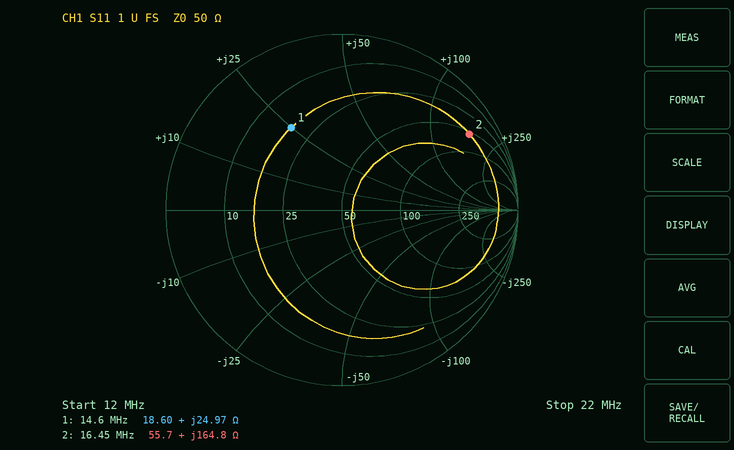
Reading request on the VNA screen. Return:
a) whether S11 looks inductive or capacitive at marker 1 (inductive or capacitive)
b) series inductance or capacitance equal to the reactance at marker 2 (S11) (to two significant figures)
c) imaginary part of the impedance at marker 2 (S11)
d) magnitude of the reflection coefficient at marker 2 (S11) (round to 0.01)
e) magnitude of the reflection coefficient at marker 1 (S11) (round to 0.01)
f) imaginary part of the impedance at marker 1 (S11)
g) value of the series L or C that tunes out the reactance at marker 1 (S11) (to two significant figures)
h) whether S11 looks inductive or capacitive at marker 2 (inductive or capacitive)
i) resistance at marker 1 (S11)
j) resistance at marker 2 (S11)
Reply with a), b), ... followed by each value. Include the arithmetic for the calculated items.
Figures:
a) inductive
b) L = 164.8 Ω/(2π × 16.45 MHz) ≈ 1.6 µH
c) +164.8 Ω
d) 0.84
e) 0.55
f) +24.97 Ω
g) C = 1/(2π × 14.6 MHz × 24.97 Ω) ≈ 437 pF, so 440 pF to two significant figures
h) inductive
i) 18.60 Ω
j) 55.7 Ω
